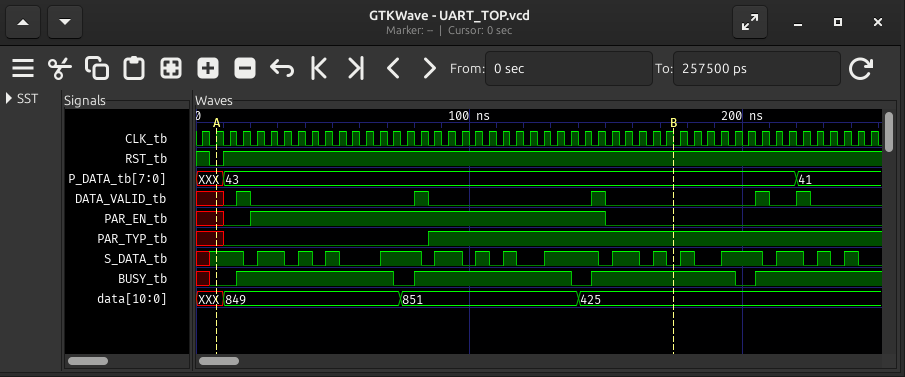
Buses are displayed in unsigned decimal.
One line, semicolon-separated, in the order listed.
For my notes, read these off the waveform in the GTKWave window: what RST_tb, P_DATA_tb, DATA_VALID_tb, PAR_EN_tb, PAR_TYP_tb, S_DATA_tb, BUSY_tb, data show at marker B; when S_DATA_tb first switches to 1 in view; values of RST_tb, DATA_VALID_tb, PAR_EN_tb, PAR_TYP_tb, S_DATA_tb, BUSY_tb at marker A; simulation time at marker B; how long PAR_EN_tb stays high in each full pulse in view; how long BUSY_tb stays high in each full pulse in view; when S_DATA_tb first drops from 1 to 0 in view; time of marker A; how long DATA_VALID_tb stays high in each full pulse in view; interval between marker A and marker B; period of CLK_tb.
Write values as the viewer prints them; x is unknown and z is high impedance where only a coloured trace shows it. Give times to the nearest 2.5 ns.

RST_tb=1, P_DATA_tb=43, DATA_VALID_tb=0, PAR_EN_tb=0, PAR_TYP_tb=1, S_DATA_tb=0, BUSY_tb=1, data=425; 5 ns; RST_tb=0, DATA_VALID_tb=x, PAR_EN_tb=x, PAR_TYP_tb=x, S_DATA_tb=1, BUSY_tb=0; 175 ns; 130 ns; 57.5 ns, 57.5 ns, 52.5 ns; 17.5 ns; 7.5 ns; 5 ns, 5 ns, 5 ns, 5 ns, 5 ns; 167.5 ns; 5 ns
